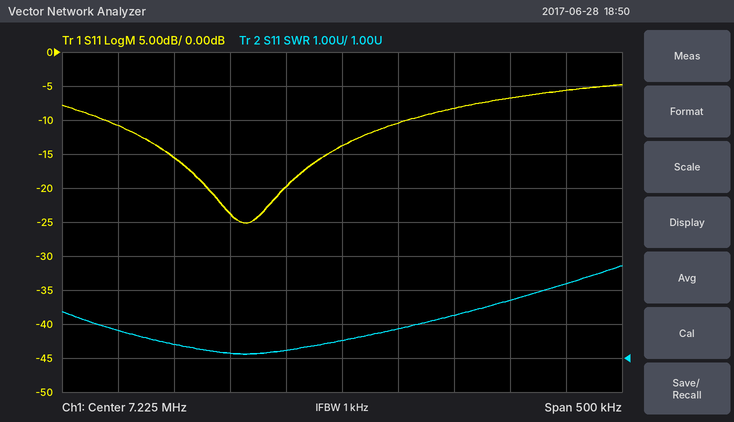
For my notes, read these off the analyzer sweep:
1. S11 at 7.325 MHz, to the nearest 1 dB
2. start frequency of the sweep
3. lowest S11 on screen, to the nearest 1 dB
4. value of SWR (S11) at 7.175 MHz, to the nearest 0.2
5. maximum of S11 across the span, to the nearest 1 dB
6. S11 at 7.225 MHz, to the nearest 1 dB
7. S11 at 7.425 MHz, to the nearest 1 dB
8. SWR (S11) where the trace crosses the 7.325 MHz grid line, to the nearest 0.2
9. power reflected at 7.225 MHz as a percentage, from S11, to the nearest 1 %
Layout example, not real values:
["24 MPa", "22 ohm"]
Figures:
["-8 dB", "6.975 MHz", "-25 dB", "1.2", "-5 dB", "-14 dB", "-6 dB", "2.2", "4 %"]
